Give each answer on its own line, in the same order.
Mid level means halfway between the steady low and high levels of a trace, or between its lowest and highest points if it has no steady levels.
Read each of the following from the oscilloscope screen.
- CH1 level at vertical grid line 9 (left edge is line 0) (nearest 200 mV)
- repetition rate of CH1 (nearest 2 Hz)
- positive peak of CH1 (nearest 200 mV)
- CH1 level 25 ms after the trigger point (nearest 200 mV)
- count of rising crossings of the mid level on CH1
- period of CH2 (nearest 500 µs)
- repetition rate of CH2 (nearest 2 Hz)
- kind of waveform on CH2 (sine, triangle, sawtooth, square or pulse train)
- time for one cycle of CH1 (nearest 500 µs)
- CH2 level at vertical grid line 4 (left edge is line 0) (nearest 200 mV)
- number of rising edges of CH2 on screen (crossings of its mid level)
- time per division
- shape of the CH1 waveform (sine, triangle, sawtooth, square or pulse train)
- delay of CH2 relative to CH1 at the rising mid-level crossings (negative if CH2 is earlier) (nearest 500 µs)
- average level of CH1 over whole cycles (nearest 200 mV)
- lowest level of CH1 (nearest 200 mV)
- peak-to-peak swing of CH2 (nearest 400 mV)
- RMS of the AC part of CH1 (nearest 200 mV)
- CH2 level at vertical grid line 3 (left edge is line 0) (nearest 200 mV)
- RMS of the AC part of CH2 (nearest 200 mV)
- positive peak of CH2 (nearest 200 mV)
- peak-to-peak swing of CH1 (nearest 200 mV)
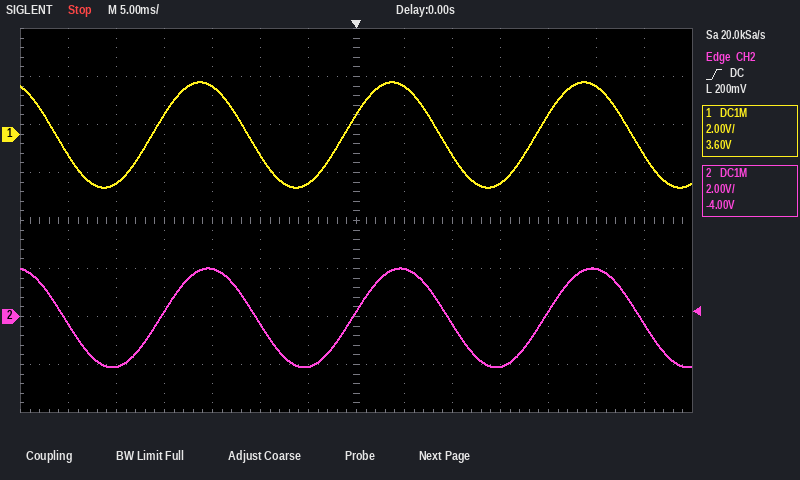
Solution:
-800 mV
50 Hz
2.2 V
2.0 V
3
20.0 ms
50 Hz
sine
20.0 ms
2.0 V
3
5 ms
sine
+1.0 ms
0.0 V
-2.2 V
4.0 V
1.6 V
200 mV
1.4 V
2.0 V
4.4 V
